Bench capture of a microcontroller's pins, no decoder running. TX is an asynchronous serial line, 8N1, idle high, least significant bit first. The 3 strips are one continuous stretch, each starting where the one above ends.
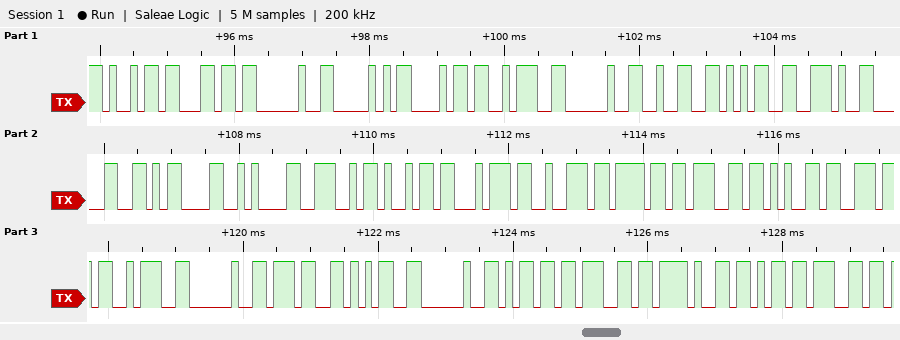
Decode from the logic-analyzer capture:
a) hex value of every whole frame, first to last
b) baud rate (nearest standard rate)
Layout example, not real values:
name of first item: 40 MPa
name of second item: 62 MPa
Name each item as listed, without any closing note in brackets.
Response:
hex value of every whole frame, first to last: 0x69 0x6C 0x20 0x50 0x68 0x3A 0x20 0x32 0x35 0x2E 0x30 0x0D 0x0A 0x4E 0x69 0x74 0x72 0x6F 0x67 0x65 0x6E 0x3A 0x20 0x37 0x35 0x20 0x6D 0x67 0x2F 0x6B 0x67
baud rate: 9600 baud
